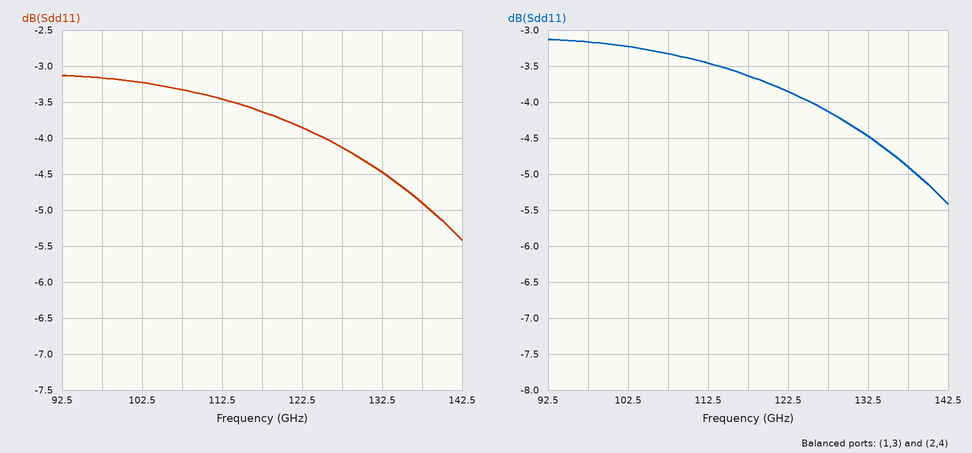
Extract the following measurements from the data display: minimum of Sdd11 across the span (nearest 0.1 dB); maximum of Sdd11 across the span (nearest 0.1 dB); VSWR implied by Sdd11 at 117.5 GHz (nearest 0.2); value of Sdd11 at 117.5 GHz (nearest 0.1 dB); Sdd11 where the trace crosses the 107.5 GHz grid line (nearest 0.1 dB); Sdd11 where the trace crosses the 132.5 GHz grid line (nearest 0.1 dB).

-5.4 dB
-3.1 dB
4.8
-3.6 dB
-3.3 dB
-4.5 dB
